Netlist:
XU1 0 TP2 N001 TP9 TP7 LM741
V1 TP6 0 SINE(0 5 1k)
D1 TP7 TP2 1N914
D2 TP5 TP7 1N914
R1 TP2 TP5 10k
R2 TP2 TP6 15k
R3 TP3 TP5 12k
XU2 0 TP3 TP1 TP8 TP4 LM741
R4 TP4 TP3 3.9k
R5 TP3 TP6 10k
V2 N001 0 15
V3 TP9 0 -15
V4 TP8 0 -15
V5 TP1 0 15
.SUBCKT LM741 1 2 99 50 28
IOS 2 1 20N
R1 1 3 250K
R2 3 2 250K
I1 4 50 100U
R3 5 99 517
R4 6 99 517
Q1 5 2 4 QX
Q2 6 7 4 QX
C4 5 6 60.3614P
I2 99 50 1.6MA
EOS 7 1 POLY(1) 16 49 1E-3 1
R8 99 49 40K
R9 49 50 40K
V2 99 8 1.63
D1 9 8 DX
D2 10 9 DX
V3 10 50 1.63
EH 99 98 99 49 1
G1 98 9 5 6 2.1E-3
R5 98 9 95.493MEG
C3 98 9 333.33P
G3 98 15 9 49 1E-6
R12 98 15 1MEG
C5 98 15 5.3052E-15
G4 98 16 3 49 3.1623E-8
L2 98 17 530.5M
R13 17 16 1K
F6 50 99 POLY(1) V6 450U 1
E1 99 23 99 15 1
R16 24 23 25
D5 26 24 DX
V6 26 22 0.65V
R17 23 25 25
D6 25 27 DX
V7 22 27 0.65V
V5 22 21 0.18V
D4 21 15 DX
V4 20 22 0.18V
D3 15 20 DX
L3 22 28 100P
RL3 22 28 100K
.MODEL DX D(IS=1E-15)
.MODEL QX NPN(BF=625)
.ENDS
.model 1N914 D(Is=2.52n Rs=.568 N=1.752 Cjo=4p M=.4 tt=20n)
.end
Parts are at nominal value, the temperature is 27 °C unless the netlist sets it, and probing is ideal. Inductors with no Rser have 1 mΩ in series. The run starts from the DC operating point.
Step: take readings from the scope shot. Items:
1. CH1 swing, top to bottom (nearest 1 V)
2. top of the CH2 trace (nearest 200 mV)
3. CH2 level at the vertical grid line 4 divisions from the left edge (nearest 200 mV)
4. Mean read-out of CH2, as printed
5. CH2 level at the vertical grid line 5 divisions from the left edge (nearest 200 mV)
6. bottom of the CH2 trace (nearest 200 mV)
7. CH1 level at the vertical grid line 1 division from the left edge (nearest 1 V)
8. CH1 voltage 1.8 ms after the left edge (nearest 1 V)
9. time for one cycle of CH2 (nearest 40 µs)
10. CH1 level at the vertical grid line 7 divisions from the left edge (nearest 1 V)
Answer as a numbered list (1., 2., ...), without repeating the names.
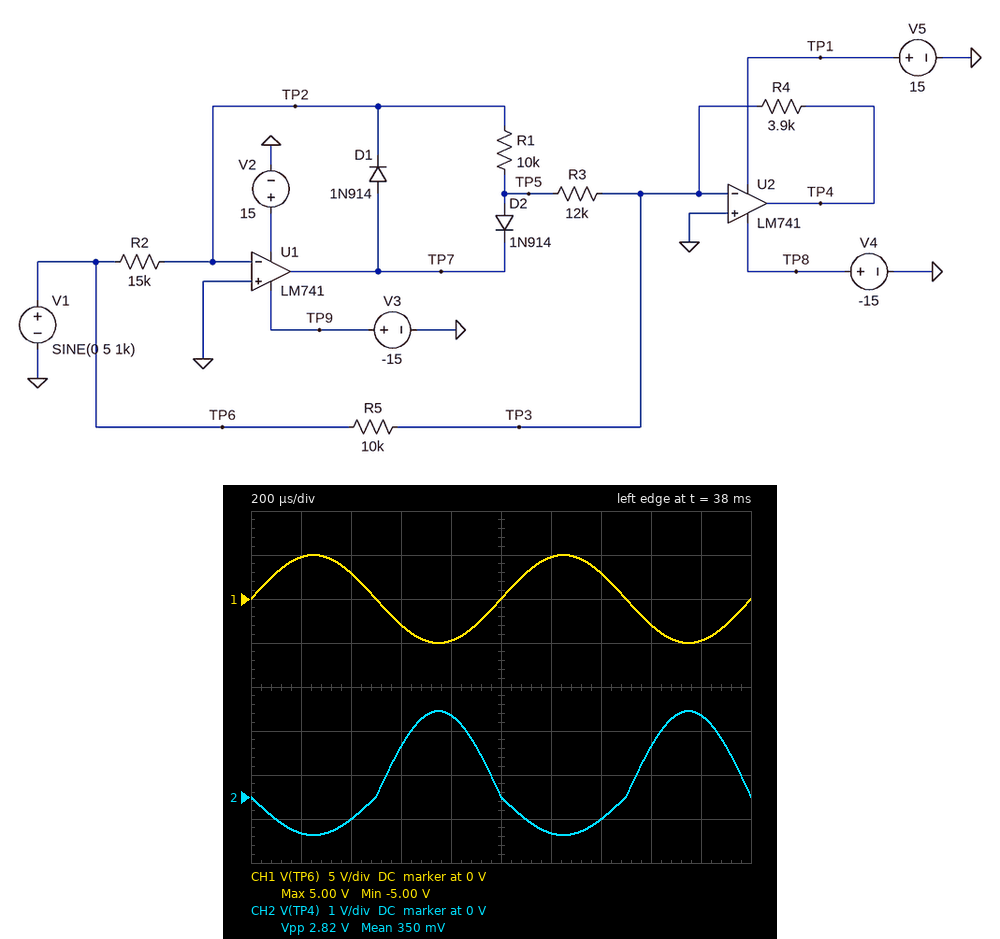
1. 10 V
2. 2.0 V
3. 1.8 V
4. 350 mV
5. 0 V
6. -800 mV
7. 5 V
8. -5 V
9. 1.00 ms
10. 3 V
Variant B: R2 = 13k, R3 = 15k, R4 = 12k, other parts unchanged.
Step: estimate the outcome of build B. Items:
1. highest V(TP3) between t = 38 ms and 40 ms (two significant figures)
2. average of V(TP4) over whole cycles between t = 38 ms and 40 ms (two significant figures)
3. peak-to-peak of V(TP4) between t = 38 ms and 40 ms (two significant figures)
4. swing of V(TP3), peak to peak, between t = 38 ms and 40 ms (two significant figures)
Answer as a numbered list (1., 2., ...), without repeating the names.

1. 8.1 mV
2. 980 mV
3. 8.9 V
4. 14 mV
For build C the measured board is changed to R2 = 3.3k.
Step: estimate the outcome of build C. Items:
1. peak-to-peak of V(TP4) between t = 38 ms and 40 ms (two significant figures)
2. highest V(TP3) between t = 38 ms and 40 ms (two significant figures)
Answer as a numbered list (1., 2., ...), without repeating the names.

1. 2.6 V
2. 4.1 mV
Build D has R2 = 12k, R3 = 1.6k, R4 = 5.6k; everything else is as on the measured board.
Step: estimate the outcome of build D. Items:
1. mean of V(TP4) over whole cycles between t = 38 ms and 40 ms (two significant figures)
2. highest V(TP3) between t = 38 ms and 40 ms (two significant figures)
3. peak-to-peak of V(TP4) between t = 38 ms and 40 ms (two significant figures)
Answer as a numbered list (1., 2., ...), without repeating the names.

1. 4.6 V
2. 13 mV
3. 12 V
